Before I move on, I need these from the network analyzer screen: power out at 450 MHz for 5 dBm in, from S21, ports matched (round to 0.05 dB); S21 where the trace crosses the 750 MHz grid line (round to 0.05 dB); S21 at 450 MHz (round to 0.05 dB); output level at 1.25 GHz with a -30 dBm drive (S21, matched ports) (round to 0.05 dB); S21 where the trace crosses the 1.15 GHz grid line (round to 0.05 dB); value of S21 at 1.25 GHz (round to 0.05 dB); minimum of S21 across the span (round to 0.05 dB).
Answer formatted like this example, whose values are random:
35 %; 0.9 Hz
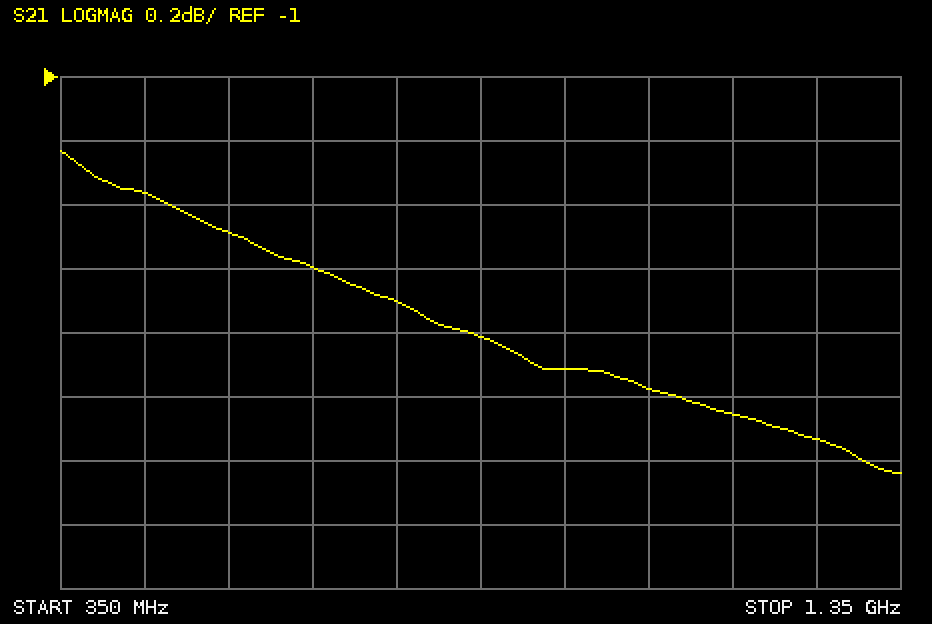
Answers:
3.65 dBm; -1.70 dB; -1.35 dB; -32.15 dBm; -2.05 dB; -2.15 dB; -2.25 dB
